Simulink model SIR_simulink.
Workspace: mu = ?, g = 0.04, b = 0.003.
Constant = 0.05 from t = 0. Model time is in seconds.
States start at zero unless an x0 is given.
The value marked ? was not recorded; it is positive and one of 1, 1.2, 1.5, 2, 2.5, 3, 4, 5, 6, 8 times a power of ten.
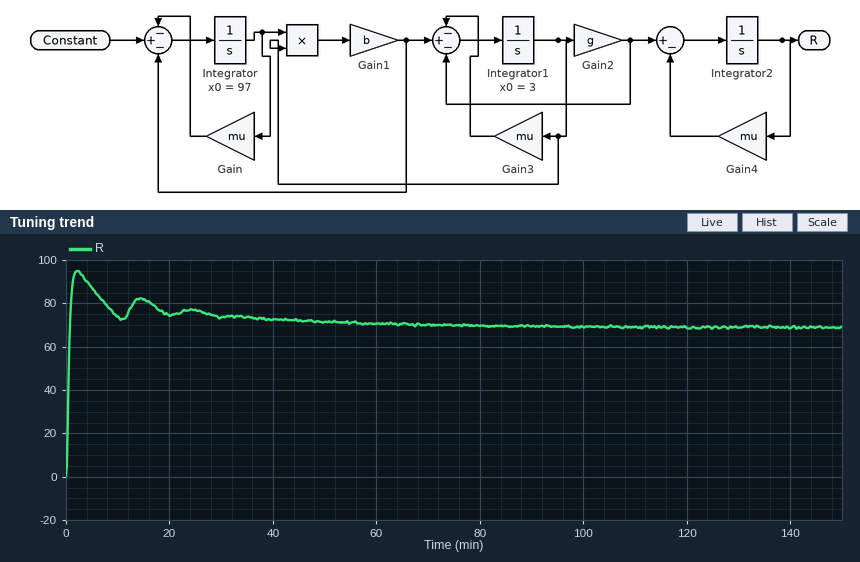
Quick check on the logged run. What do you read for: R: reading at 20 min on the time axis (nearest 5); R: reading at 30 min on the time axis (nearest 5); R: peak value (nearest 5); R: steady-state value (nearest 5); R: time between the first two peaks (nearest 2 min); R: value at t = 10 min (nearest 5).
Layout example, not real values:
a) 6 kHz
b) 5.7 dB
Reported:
a) 75
b) 75
c) 95
d) 70
e) 12 min
f) 75
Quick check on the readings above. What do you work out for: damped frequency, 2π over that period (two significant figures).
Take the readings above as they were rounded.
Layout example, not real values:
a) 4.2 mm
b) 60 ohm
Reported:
a) 0.52 rad/min
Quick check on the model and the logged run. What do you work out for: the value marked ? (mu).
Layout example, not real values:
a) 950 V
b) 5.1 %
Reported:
a) 0.0006
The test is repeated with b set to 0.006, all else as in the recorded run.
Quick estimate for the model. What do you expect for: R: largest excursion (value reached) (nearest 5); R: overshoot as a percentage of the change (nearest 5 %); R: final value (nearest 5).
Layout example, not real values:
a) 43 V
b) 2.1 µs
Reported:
a) 95
b) 25 %
c) 75
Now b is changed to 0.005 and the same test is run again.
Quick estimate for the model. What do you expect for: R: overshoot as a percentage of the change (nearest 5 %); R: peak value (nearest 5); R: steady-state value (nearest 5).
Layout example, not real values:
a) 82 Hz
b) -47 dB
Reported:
a) 30 %
b) 95
c) 75
